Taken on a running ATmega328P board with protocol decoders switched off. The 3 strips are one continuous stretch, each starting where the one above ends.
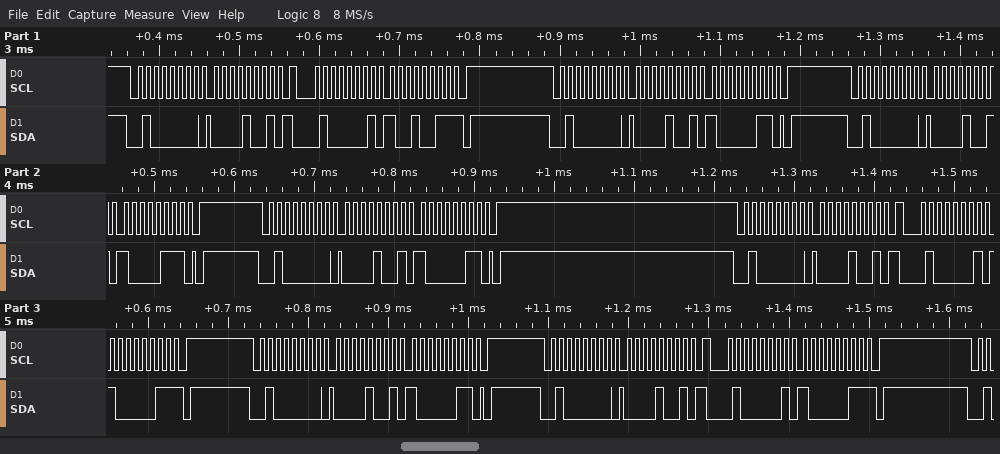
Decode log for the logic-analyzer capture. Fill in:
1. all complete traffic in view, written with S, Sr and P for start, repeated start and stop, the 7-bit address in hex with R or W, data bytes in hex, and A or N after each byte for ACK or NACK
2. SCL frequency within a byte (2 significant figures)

S 20W A 09 A Sr 20R A 93 N P S 20W A 09 A 83 A P S 20W A 09 A 87 A P S 20W A 09 A 83 A P S 20W A 09 A Sr 20R A 83 N P S 20W A 09 A 83 A P S 20W A 09 A Sr 20R A 83 N P
100 kHz
